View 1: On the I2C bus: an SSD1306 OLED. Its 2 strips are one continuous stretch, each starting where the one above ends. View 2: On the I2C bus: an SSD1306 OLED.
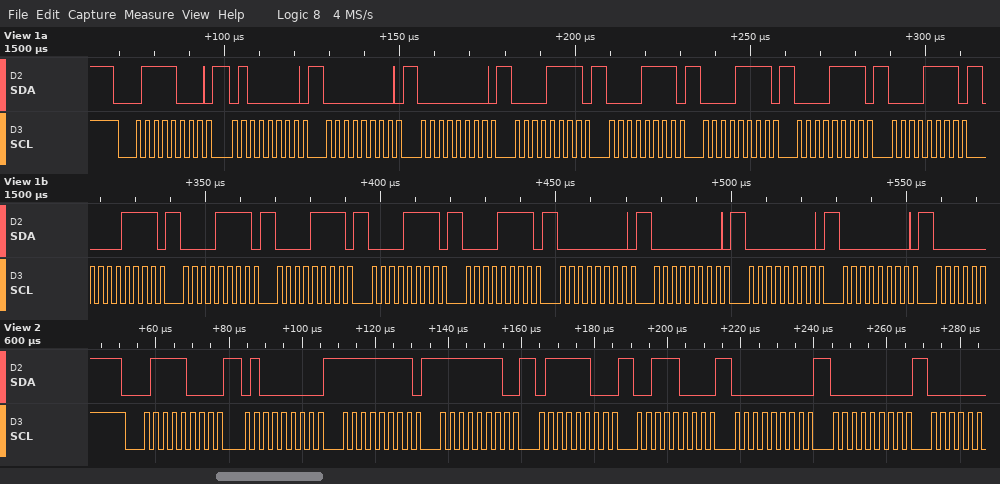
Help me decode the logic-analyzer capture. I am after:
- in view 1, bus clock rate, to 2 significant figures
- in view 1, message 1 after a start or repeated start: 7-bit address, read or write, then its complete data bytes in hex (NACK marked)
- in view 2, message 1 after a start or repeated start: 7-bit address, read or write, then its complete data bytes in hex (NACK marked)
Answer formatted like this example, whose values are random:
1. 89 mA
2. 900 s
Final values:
1. 400 kHz
2. 0x3C write: 40 00 00 0F 0F 0F 0F 0F 0F 0F 0F 0F 0F 00 00 00 00
3. 0x3C write: 40 FF FE 7C 38 00 00
